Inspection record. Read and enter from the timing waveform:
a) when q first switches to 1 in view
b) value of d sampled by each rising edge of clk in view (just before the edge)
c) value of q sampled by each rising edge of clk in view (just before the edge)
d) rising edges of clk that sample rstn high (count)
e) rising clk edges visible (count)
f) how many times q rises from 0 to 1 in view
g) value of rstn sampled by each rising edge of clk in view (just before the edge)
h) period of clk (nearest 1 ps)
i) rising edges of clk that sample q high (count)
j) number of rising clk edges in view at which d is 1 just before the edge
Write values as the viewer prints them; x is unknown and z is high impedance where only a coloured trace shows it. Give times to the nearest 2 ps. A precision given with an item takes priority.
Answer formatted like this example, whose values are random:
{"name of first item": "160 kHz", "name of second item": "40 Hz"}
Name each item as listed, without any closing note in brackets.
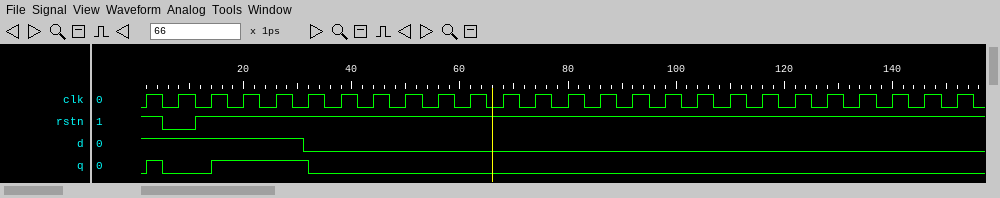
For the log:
{"when q first switches to 1 in view": "2 ps", "value of d sampled by each rising edge of clk in view": "1 1 1 1 1 0 0 0 0 0 0 0 0 0 0 0 0 0 0 0 0 0 0 0 0 0", "value of q sampled by each rising edge of clk in view": "0 0 0 1 1 1 0 0 0 0 0 0 0 0 0 0 0 0 0 0 0 0 0 0 0 0", "rising edges of clk that sample rstn high": "25", "rising clk edges visible": "26", "how many times q rises from 0 to 1 in view": "2", "value of rstn sampled by each rising edge of clk in view": "1 0 1 1 1 1 1 1 1 1 1 1 1 1 1 1 1 1 1 1 1 1 1 1 1 1", "period of clk": "6 ps", "rising edges of clk that sample q high": "3", "number of rising clk edges in view at which d is 1 just before the edge": "5"}
